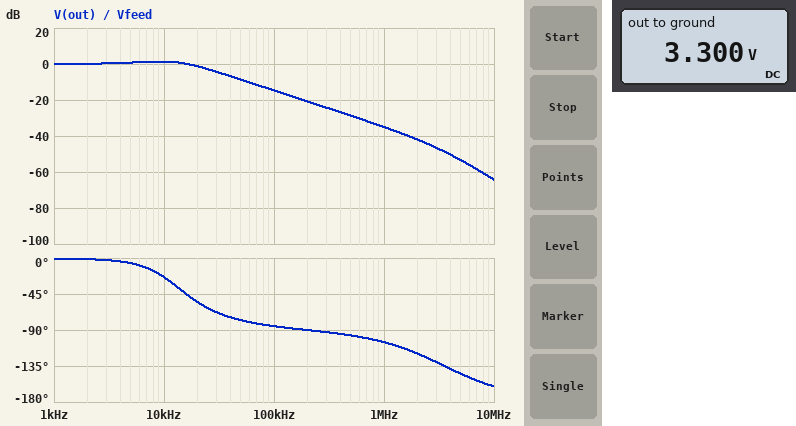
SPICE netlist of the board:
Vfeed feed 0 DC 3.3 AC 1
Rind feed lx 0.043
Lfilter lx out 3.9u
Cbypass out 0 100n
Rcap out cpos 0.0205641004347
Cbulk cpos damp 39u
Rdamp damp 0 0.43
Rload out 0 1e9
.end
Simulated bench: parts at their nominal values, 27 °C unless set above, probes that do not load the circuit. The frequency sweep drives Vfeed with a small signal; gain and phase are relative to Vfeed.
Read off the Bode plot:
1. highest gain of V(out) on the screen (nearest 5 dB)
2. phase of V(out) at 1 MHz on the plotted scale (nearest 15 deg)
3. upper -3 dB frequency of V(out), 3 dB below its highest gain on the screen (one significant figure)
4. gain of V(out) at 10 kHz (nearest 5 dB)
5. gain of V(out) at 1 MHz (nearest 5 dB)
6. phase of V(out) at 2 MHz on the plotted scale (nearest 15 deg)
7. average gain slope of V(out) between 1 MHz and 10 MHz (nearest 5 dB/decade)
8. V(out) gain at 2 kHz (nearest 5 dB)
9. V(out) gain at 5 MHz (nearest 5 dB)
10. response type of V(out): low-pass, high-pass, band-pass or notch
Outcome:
0 dB
-105 deg
20 kHz
0 dB
-35 dB
-120 deg
-30 dB/decade
0 dB
-55 dB
low-pass
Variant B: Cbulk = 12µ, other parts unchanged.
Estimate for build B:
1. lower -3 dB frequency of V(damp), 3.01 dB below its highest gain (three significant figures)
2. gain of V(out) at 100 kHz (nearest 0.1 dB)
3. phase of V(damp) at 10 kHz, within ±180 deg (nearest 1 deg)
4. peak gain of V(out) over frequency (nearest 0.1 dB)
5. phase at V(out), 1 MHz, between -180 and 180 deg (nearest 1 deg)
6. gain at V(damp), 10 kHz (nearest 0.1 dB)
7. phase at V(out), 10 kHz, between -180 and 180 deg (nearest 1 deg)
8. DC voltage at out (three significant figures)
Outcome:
15.3 kHz
-14.1 dB
65 deg
3.8 dB
-106 deg
-8.8 dB
-6 deg
3.30 V
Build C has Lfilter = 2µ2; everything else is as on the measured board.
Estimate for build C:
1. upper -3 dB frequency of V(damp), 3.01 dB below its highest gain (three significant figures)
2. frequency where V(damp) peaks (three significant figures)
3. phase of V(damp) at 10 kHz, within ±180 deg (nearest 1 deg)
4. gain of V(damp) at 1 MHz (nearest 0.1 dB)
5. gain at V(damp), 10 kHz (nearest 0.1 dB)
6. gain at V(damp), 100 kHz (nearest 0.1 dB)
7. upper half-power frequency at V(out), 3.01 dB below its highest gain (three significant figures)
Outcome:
42.8 kHz
17.2 kHz
29 deg
-30.4 dB
-2.3 dB
-10.4 dB
34.6 kHz
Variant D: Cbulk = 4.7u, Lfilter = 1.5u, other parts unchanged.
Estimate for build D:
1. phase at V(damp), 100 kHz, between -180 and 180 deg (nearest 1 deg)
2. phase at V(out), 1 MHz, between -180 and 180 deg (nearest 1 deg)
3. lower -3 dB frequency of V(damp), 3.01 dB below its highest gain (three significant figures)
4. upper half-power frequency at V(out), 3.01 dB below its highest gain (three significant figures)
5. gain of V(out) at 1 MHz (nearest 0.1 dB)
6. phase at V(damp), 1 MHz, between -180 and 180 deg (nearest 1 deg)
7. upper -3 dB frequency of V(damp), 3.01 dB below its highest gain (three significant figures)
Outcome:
-53 deg
-107 deg
39.4 kHz
77.6 kHz
-26.8 dB
-103 deg
90.4 kHz
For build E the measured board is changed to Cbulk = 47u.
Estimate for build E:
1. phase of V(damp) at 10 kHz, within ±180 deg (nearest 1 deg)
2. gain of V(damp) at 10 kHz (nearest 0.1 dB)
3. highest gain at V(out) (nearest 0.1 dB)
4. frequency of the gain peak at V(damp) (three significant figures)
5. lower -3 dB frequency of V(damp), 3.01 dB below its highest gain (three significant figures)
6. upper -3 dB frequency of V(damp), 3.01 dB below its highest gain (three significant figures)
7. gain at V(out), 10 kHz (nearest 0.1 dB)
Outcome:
11 deg
-1.3 dB
1.1 dB
11.8 kHz
5.42 kHz
25.6 kHz
1.0 dB
